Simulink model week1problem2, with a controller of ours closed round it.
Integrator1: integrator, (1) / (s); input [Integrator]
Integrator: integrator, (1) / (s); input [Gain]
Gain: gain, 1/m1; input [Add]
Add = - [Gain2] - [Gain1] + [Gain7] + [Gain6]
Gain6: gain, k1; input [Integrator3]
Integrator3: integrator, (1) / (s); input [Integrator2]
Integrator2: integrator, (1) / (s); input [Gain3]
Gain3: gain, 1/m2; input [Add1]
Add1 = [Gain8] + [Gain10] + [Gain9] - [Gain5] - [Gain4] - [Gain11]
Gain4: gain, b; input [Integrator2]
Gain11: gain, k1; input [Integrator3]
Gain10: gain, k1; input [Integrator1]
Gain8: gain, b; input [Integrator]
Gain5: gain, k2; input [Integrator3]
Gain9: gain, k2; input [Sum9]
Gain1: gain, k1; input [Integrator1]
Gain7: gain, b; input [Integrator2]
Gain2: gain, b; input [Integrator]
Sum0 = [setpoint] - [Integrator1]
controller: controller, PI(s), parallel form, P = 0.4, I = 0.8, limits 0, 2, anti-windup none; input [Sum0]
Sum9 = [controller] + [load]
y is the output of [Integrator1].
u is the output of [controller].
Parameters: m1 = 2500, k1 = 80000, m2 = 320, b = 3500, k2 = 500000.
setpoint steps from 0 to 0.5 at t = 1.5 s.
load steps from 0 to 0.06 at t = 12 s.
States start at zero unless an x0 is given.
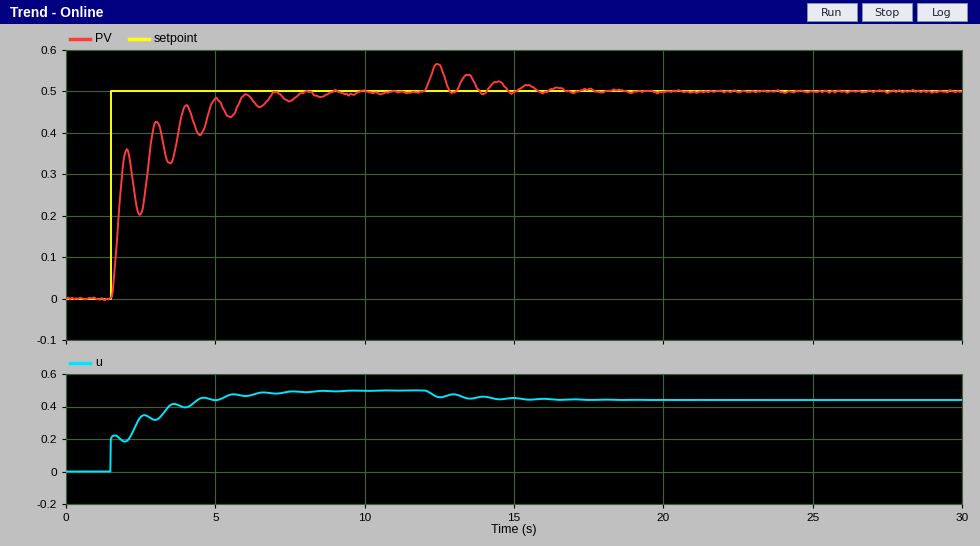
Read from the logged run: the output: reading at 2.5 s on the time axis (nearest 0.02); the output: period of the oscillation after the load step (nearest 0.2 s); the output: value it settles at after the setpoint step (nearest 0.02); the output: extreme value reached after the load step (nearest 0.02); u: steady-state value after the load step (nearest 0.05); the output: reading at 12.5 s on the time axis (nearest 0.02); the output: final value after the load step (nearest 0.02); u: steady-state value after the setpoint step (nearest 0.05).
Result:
0.20
1.0 s
0.50
0.56
0.45
0.56
0.50
0.50
